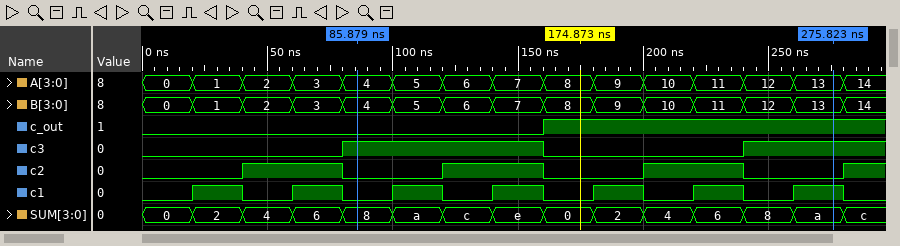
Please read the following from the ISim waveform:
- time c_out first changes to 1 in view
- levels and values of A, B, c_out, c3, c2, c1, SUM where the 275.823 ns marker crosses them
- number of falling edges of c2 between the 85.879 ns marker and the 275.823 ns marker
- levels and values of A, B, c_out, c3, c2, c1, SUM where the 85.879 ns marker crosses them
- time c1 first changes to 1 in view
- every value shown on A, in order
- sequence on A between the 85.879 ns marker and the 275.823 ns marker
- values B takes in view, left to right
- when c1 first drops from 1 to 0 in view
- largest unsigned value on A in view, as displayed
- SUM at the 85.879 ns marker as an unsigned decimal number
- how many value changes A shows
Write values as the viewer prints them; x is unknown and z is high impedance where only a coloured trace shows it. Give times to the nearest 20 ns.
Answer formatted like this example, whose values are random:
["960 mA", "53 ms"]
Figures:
["160 ns", "A=13, B=13, c_out=1, c3=1, c2=0, c1=1, SUM=a", "2", "A=4, B=4, c_out=0, c3=1, c2=0, c1=0, SUM=8", "20 ns", "0, 1, 2, 3, 4, 5, 6, 7, 8, 9, 10, 11, 12, 13, 14", "4, 5, 6, 7, 8, 9, 10, 11, 12, 13", "0, 1, 2, 3, 4, 5, 6, 7, 8, 9, 10, 11, 12, 13, 14", "40 ns", "14", "8", "14"]
